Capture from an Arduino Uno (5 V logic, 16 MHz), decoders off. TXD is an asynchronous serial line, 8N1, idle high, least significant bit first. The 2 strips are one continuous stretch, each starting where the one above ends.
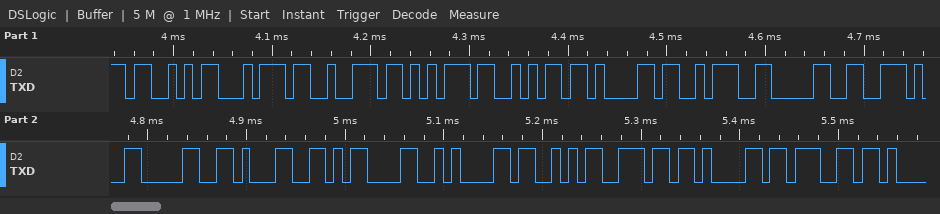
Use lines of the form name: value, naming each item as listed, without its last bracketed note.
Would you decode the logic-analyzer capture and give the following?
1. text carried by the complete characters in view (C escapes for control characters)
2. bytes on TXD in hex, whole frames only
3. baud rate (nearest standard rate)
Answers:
text carried by the complete characters in view: "Struja:0.01\r\nSnag"
bytes on TXD in hex, whole frames only: 53 74 72 75 6A 61 3A 30 2E 30 31 0D 0A 53 6E 61 67
baud rate: 115200 baud
